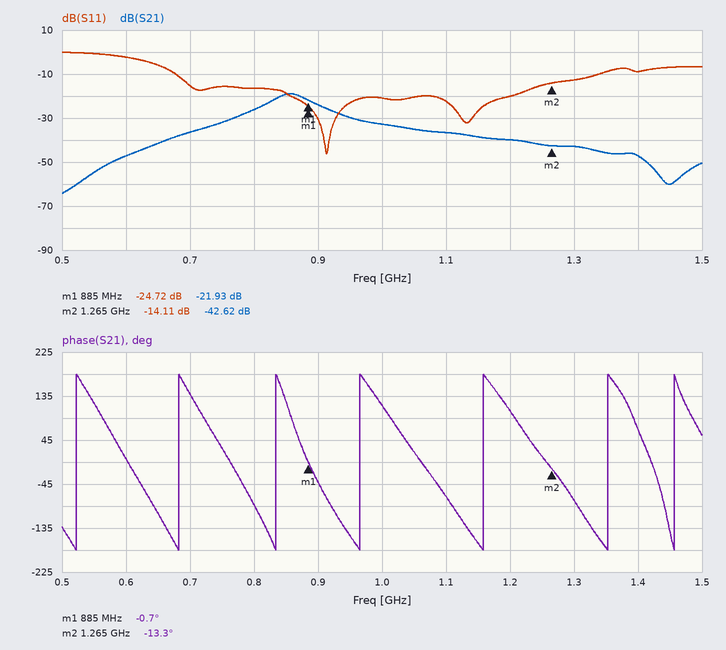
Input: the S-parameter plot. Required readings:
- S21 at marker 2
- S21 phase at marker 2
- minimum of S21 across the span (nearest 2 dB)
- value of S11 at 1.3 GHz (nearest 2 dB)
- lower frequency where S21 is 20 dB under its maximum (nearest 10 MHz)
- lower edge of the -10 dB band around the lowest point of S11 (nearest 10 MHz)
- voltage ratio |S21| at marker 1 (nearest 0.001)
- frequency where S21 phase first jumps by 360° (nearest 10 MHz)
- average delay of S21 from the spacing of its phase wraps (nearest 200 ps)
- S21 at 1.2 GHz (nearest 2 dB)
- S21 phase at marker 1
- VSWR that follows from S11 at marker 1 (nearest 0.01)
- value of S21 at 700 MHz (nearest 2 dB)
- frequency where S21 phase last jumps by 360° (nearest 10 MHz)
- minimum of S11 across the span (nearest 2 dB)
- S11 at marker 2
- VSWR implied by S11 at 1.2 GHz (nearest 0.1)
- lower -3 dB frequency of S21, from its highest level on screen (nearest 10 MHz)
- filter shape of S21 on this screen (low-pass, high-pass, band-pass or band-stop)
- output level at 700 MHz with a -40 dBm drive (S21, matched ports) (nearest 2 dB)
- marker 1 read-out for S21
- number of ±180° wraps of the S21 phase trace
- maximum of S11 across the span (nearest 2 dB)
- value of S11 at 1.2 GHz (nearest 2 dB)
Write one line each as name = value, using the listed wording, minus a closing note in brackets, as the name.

S21 at marker 2 = -42.62 dB
S21 phase at marker 2 = -13.3°
minimum of S21 across the span = -64 dB
value of S11 at 1.3 GHz = -12 dB
lower frequency where S21 is 20 dB under its maximum = 670 MHz
lower edge of the -10 dB band around the lowest point of S11 = 680 MHz
voltage ratio |S21| at marker 1 = 0.080
frequency where S21 phase first jumps by 360° = 520 MHz
average delay of S21 from the spacing of its phase wraps = 6.4 ns
S21 at 1.2 GHz = -40 dB
S21 phase at marker 1 = -0.7°
VSWR that follows from S11 at marker 1 = 1.12
value of S21 at 700 MHz = -36 dB
frequency where S21 phase last jumps by 360° = 1.46 GHz
minimum of S11 across the span = -46 dB
S11 at marker 2 = -14.11 dB
VSWR implied by S11 at 1.2 GHz = 1.2
lower -3 dB frequency of S21, from its highest level on screen = 830 MHz
filter shape of S21 on this screen = band-pass
output level at 700 MHz with a -40 dBm drive (S21, matched ports) = -76 dBm
marker 1 read-out for S21 = -21.93 dB
number of ±180° wraps of the S21 phase trace = 7
maximum of S11 across the span = 0 dB
value of S11 at 1.2 GHz = -20 dB
